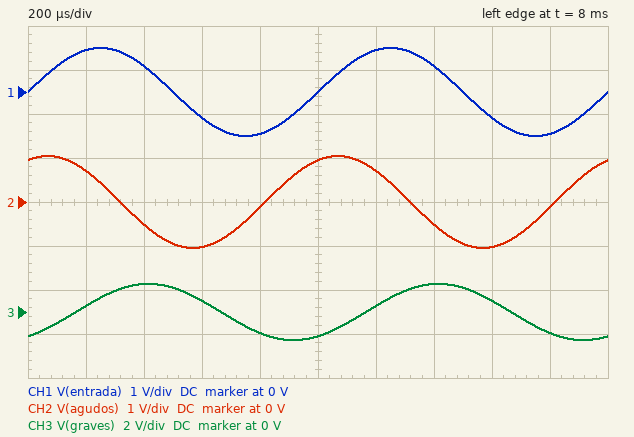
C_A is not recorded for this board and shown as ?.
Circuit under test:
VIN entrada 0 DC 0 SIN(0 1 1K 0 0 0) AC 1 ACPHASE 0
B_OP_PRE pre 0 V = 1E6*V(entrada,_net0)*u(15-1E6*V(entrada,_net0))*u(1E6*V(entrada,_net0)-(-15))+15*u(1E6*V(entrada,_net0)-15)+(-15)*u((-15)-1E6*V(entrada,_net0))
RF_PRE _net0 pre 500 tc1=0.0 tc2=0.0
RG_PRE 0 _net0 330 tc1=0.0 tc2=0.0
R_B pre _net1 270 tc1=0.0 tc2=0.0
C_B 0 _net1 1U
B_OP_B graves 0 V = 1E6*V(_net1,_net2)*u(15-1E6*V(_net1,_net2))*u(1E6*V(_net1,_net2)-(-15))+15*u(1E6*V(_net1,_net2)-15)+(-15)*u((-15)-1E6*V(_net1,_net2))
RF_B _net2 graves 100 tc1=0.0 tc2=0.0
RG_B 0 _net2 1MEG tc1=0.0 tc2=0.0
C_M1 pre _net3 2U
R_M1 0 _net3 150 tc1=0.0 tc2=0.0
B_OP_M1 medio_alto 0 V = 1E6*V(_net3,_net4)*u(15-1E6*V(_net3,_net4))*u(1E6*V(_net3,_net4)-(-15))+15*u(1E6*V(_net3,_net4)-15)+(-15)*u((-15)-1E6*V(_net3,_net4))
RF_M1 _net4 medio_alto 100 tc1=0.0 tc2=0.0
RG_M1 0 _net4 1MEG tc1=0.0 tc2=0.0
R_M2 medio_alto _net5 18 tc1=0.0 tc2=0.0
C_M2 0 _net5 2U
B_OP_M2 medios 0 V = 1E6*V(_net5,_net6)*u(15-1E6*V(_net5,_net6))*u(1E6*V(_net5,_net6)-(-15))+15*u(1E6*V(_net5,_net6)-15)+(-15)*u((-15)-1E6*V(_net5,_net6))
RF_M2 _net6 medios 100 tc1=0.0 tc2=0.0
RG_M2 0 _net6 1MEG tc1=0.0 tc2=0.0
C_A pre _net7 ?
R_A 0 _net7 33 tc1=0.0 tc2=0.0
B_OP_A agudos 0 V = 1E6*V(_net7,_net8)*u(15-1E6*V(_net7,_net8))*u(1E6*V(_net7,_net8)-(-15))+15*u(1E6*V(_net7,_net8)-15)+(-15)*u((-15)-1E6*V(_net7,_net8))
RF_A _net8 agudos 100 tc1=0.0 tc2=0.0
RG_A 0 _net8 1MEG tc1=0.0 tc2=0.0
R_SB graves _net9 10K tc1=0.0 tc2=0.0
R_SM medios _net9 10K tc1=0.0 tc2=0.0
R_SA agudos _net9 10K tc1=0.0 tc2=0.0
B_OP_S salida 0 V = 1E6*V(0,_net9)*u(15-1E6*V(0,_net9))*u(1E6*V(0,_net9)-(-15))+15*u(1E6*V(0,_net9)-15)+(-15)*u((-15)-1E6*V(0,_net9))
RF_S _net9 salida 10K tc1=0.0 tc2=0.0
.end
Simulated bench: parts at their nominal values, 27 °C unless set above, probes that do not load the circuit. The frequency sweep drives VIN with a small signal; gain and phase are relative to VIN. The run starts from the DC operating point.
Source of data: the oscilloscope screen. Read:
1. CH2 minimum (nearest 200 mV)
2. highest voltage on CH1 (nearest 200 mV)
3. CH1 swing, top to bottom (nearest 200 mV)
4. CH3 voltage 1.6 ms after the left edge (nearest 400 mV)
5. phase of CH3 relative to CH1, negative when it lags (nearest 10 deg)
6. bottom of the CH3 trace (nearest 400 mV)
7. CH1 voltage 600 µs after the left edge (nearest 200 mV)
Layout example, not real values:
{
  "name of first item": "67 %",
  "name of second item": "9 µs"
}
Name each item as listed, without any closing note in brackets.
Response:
{
  "CH2 minimum": "-1.0 V",
  "highest voltage on CH1": "1.0 V",
  "CH1 swing, top to bottom": "2.0 V",
  "CH3 voltage 1.6 ms after the left edge": "400 mV",
  "phase of CH3 relative to CH1, negative when it lags": "-60 deg",
  "bottom of the CH3 trace": "-1.2 V",
  "CH1 voltage 600 µs after the left edge": "-600 mV"
}
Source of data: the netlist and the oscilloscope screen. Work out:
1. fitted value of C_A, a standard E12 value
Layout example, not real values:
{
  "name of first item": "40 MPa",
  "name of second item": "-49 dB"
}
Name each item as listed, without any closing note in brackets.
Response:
{
  "fitted value of C_A, a standard E12 value": "2.2 µF"
}
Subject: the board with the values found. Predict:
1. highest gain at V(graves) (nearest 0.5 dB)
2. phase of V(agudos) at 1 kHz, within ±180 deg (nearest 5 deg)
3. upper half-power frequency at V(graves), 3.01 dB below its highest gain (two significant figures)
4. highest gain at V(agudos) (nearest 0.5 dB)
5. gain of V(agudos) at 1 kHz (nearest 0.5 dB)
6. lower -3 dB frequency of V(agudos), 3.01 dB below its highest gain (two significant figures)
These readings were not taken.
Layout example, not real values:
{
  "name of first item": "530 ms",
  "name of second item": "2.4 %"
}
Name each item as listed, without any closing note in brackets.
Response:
{
  "highest gain at V(graves)": "8.0 dB",
  "phase of V(agudos) at 1 kHz, within ±180 deg": "65 deg",
  "upper half-power frequency at V(graves), 3.01 dB below its highest gain": "590 Hz",
  "highest gain at V(agudos)": "8.0 dB",
  "gain of V(agudos) at 1 kHz": "0.5 dB",
  "lower -3 dB frequency of V(agudos), 3.01 dB below its highest gain": "2.2 kHz"
}
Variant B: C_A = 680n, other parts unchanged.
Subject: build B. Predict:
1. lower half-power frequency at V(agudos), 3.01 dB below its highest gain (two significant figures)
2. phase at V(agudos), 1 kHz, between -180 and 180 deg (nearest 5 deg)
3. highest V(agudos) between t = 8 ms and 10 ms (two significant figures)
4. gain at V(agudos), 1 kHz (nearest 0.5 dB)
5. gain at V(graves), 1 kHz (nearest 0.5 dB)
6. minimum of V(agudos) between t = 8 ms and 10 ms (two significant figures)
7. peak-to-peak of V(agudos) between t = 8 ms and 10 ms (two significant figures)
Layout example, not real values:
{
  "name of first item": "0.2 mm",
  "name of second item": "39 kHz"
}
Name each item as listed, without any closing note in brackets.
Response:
{
  "lower half-power frequency at V(agudos), 3.01 dB below its highest gain": "7.1 kHz",
  "phase at V(agudos), 1 kHz, between -180 and 180 deg": "80 deg",
  "highest V(agudos) between t = 8 ms and 10 ms": "350 mV",
  "gain at V(agudos), 1 kHz": "-9.0 dB",
  "gain at V(graves), 1 kHz": "2.0 dB",
  "minimum of V(agudos) between t = 8 ms and 10 ms": "-350 mV",
  "peak-to-peak of V(agudos) between t = 8 ms and 10 ms": "700 mV"
}
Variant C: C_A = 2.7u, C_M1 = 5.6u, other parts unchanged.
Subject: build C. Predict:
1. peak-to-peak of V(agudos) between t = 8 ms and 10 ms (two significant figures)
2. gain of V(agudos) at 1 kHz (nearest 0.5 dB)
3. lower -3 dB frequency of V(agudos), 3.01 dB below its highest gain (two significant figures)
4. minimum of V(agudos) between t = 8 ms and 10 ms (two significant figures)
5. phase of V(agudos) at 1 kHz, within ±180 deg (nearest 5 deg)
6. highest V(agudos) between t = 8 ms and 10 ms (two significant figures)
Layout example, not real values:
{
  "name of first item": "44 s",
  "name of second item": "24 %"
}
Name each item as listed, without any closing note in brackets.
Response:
{
  "peak-to-peak of V(agudos) between t = 8 ms and 10 ms": "2.5 V",
  "gain of V(agudos) at 1 kHz": "2.0 dB",
  "lower -3 dB frequency of V(agudos), 3.01 dB below its highest gain": "1.8 kHz",
  "minimum of V(agudos) between t = 8 ms and 10 ms": "-1.2 V",
  "phase of V(agudos) at 1 kHz, within ±180 deg": "60 deg",
  "highest V(agudos) between t = 8 ms and 10 ms": "1.2 V"
}
